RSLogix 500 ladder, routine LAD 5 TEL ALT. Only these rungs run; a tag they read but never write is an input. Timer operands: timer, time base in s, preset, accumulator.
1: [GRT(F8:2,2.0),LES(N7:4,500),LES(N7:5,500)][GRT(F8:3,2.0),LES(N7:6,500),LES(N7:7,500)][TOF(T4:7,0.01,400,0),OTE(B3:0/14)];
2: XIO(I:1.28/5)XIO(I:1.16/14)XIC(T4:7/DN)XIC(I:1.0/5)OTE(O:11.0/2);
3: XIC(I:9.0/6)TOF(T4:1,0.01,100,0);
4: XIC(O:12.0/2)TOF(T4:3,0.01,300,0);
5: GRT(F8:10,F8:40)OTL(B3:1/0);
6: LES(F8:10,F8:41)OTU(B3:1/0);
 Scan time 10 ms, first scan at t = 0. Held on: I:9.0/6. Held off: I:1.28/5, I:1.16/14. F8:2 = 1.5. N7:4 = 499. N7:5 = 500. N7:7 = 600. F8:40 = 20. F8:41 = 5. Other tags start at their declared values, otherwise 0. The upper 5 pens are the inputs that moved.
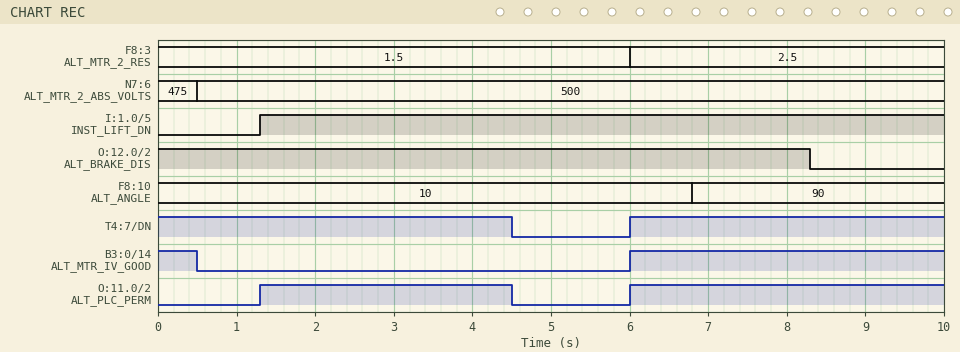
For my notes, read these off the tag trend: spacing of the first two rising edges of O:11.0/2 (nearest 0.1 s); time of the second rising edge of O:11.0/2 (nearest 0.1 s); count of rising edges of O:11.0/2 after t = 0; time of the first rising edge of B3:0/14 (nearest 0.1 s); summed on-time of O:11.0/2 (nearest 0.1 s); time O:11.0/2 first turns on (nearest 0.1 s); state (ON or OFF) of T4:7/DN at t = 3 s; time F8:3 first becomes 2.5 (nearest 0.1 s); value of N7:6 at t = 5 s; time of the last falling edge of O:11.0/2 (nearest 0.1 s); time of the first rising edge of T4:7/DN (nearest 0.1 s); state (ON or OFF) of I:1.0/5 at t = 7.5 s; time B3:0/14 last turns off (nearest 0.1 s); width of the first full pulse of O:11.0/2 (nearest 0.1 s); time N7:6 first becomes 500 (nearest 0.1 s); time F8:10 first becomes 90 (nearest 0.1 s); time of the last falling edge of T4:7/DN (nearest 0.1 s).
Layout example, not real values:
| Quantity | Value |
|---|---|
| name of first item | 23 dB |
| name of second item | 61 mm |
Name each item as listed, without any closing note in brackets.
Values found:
| Quantity | Value |
|---|---|
| spacing of the first two rising edges of O:11.0/2 | 4.7 s |
| time of the second rising edge of O:11.0/2 | 6.0 s |
| count of rising edges of O:11.0/2 after t = 0 | 2 |
| time of the first rising edge of B3:0/14 | 6.0 s |
| summed on-time of O:11.0/2 | 7.2 s |
| time O:11.0/2 first turns on | 1.3 s |
| state (ON or OFF) of T4:7/DN at t = 3 s | ON |
| time F8:3 first becomes 2.5 | 6.0 s |
| value of N7:6 at t = 5 s | 500 |
| time of the last falling edge of O:11.0/2 | 4.5 s |
| time of the first rising edge of T4:7/DN | 6.0 s |
| state (ON or OFF) of I:1.0/5 at t = 7.5 s | ON |
| time B3:0/14 last turns off | 0.5 s |
| width of the first full pulse of O:11.0/2 | 3.2 s |
| time N7:6 first becomes 500 | 0.5 s |
| time F8:10 first becomes 90 | 6.8 s |
| time of the last falling edge of T4:7/DN | 4.5 s |
